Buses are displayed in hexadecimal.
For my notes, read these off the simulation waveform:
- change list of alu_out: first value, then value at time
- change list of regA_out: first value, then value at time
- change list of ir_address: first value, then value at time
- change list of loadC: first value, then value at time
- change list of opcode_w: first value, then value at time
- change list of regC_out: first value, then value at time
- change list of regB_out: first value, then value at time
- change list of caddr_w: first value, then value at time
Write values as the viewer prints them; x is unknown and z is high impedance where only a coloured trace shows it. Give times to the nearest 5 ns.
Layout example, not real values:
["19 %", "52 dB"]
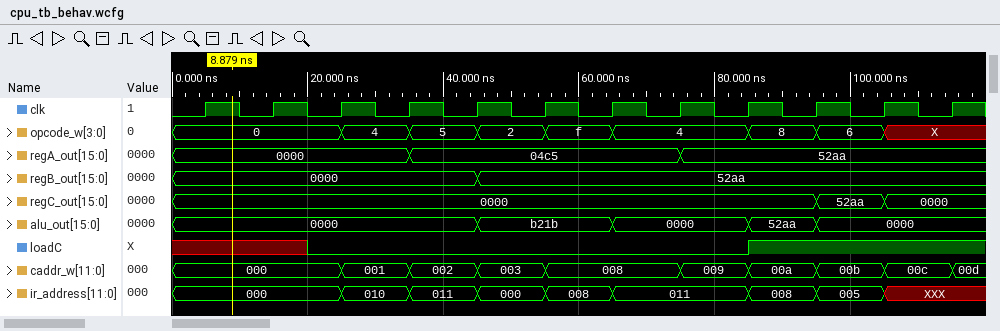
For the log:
["0000, b21b at 45 ns, 0000 at 65 ns, 52aa at 85 ns, 0000 at 95 ns", "0000, 04c5 at 35 ns, 52aa at 75 ns", "000, 010 at 25 ns, 011 at 35 ns, 000 at 45 ns, 008 at 55 ns, 011 at 65 ns, 008 at 85 ns, 005 at 95 ns, XXX at 105 ns", "x, 0 at 20 ns, 1 at 85 ns", "0, 4 at 25 ns, 5 at 35 ns, 2 at 45 ns, f at 55 ns, 4 at 65 ns, 8 at 85 ns, 6 at 95 ns, X at 105 ns", "0000, 52aa at 95 ns, 0000 at 105 ns", "0000, 52aa at 45 ns", "000, 001 at 25 ns, 002 at 35 ns, 003 at 45 ns, 008 at 55 ns, 009 at 75 ns, 00a at 85 ns, 00b at 95 ns, 00c at 105 ns, 00d at 115 ns"]
